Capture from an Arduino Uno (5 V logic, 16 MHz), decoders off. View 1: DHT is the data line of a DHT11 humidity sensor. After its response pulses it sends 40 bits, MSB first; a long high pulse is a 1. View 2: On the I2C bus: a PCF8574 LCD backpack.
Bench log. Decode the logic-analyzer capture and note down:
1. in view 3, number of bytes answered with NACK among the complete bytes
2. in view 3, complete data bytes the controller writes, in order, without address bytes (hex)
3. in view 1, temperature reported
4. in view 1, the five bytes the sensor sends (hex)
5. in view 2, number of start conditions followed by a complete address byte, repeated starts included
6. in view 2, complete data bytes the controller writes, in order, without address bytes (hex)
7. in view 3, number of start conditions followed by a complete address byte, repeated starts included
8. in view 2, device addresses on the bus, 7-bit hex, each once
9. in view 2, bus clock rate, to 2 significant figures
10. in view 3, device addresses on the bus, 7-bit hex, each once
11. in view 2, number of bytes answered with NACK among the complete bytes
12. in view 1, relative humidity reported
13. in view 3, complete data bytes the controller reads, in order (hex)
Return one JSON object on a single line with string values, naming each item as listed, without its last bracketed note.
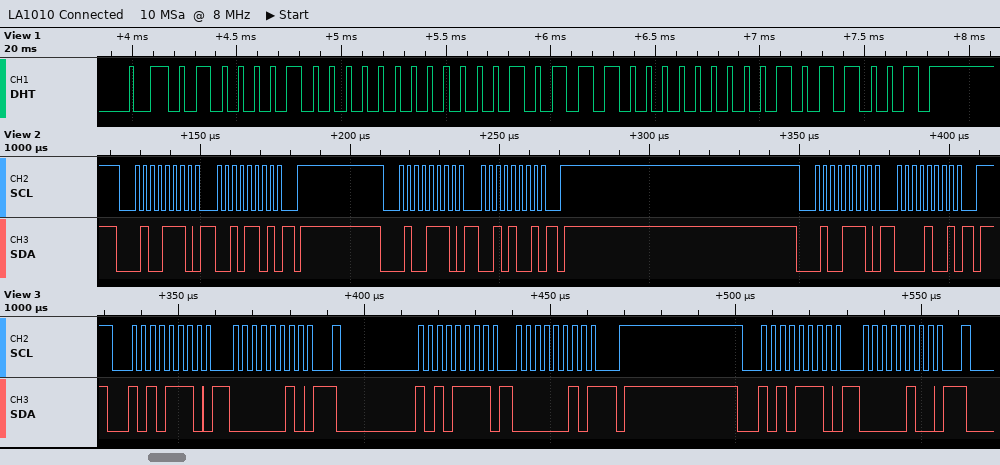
{"in view 3, number of bytes answered with NACK among the complete bytes": "1", "in view 3, complete data bytes the controller writes, in order, without address bytes": "02 04", "in view 1, temperature reported": "23.0 °C", "in view 1, the five bytes the sensor sends": "42 00 17 00 59", "in view 2, number of start conditions followed by a complete address byte, repeated starts included": "3", "in view 2, complete data bytes the controller writes, in order, without address bytes": "2D 29 09", "in view 3, number of start conditions followed by a complete address byte, repeated starts included": "3", "in view 2, device addresses on the bus, 7-bit hex, each once": "0x27", "in view 2, bus clock rate, to 2 significant figures": "400 kHz", "in view 3, device addresses on the bus, 7-bit hex, each once": "0x57", "in view 2, number of bytes answered with NACK among the complete bytes": "0", "in view 1, relative humidity reported": "66 %", "in view 3, complete data bytes the controller reads, in order": "02"}
